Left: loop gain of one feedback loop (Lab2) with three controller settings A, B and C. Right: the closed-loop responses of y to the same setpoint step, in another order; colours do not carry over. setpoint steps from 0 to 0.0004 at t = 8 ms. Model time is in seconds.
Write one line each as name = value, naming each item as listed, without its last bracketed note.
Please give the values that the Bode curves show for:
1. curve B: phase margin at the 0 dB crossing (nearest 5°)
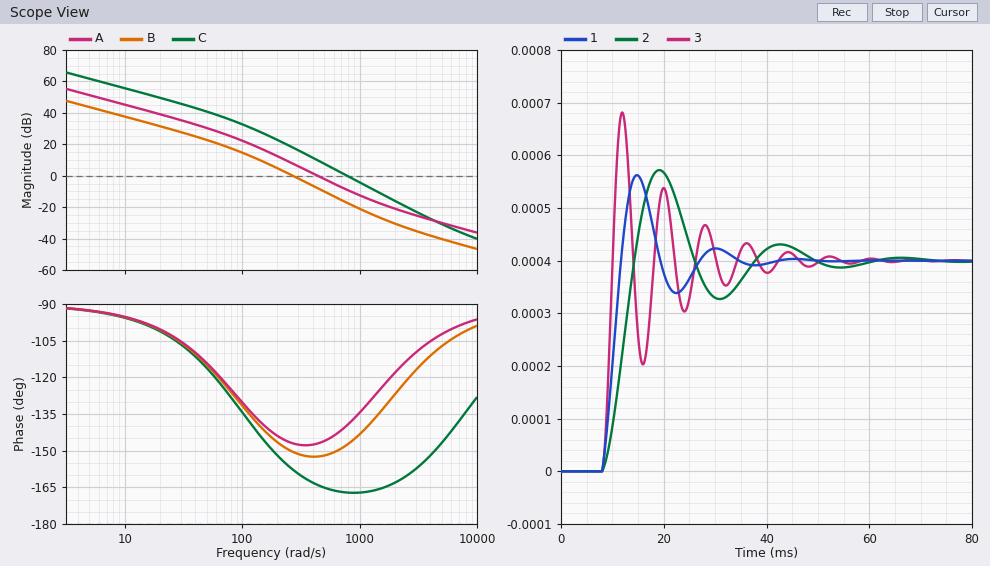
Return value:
curve B: phase margin at the 0 dB crossing = 30°
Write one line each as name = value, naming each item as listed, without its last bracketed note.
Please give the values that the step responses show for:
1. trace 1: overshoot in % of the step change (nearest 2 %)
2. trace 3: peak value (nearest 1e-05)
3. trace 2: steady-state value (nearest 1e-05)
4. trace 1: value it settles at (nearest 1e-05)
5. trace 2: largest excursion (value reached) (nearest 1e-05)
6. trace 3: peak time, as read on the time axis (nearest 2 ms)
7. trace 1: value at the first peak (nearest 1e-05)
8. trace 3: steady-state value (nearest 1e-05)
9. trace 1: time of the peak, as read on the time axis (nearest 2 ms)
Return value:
trace 1: overshoot in % of the step change = 40 %
trace 3: peak value = 0.00068
trace 2: steady-state value = 0.00040
trace 1: value it settles at = 0.00040
trace 2: largest excursion (value reached) = 0.00057
trace 3: peak time, as read on the time axis = 12 ms
trace 1: value at the first peak = 0.00056
trace 3: steady-state value = 0.00040
trace 1: time of the peak, as read on the time axis = 14 ms
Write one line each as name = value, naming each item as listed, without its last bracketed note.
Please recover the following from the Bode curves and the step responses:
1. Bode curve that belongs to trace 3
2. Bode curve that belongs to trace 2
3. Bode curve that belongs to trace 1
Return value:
Bode curve that belongs to trace 3 = C
Bode curve that belongs to trace 2 = B
Bode curve that belongs to trace 1 = A
